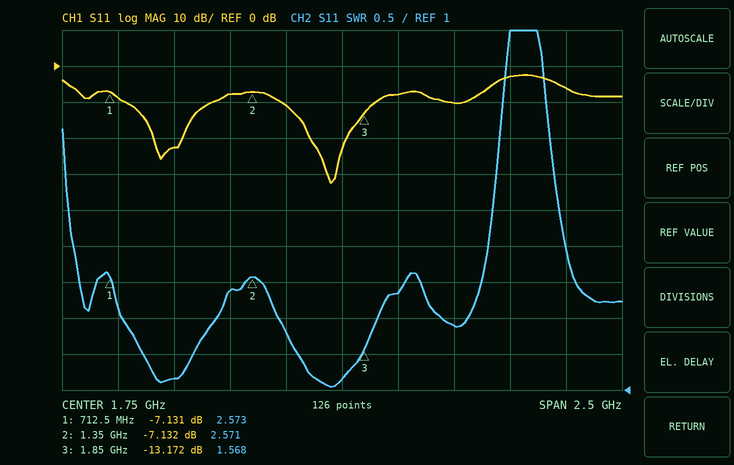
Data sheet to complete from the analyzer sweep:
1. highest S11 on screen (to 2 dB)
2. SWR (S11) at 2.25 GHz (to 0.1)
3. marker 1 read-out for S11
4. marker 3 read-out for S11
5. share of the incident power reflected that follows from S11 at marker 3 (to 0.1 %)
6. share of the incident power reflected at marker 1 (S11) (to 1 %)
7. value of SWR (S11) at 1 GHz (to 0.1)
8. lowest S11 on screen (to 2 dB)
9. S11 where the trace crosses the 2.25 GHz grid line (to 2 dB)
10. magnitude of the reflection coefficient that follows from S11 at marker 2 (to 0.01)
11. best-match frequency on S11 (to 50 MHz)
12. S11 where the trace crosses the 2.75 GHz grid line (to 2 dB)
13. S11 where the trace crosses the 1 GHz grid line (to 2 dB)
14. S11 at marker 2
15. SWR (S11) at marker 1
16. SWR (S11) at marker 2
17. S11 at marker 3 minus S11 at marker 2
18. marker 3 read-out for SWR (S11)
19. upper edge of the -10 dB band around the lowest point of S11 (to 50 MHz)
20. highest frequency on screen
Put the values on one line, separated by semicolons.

-2 dB; 1.9; -7.131 dB; -13.172 dB; 4.8 %; 19 %; 1.2; -32 dB; -10 dB; 0.44; 1.70 GHz; -6 dB; -22 dB; -7.132 dB; 2.573; 2.571; -6.040 dB; 1.568; 1.90 GHz; 3 GHz
